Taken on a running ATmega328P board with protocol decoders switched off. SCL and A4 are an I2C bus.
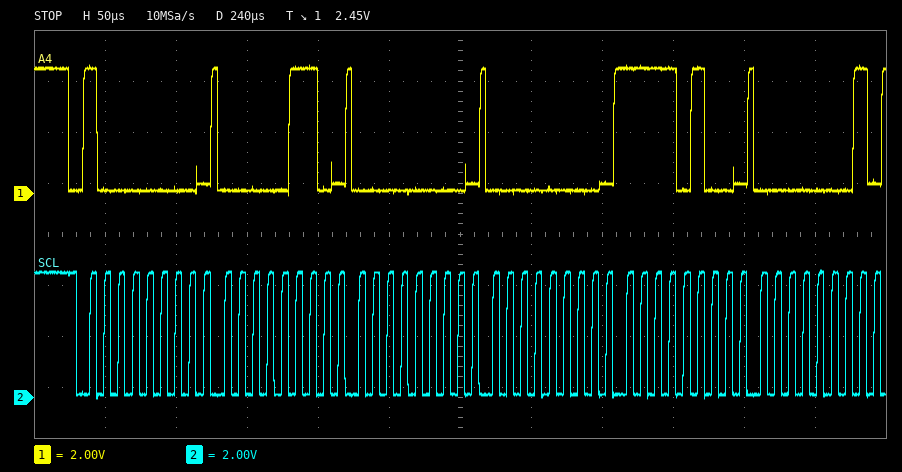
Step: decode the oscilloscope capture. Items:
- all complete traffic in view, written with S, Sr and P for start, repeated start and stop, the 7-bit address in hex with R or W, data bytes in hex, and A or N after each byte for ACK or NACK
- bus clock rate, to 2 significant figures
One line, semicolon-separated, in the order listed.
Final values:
S 40W A 06 A 00 A 00 A F4 A 01 A; 100 kHz
